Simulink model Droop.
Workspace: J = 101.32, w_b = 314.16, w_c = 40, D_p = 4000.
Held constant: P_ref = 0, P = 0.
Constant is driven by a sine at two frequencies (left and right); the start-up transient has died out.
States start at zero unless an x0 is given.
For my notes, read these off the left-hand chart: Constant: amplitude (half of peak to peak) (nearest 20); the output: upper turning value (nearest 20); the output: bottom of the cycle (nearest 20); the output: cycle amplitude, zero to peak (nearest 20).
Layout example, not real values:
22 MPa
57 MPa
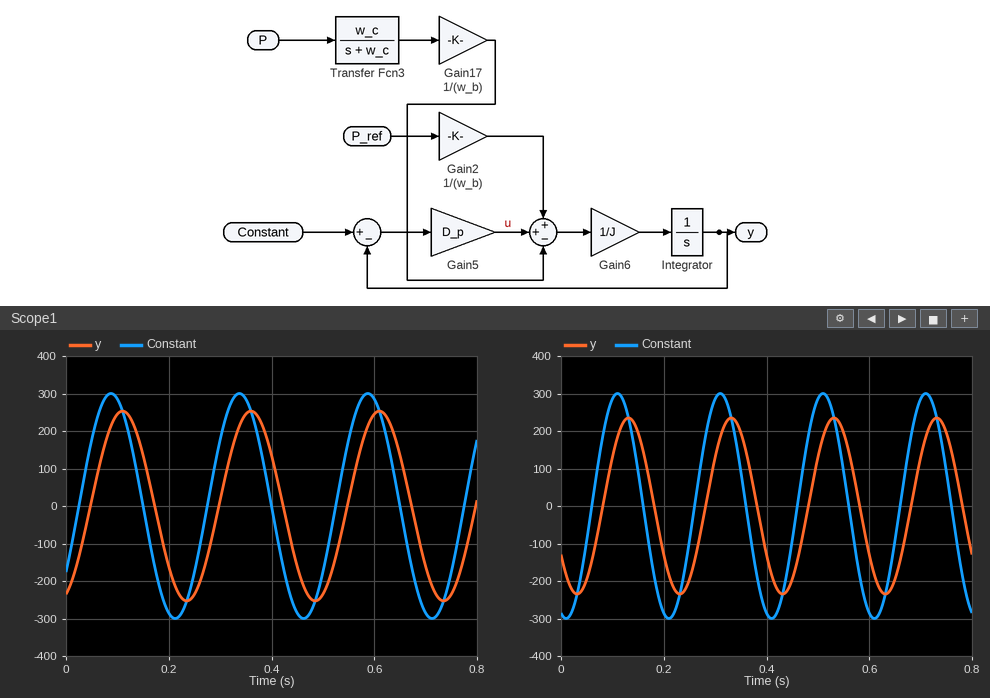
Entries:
300
260
-260
260
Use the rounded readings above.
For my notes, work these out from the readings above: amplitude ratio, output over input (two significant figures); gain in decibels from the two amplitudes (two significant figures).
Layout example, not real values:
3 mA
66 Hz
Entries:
0.87
-1.2 dB
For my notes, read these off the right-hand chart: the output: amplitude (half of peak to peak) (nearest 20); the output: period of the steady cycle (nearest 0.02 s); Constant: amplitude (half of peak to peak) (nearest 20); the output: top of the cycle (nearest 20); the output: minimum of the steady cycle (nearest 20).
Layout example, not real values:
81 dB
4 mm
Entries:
240
0.20 s
300
240
-240
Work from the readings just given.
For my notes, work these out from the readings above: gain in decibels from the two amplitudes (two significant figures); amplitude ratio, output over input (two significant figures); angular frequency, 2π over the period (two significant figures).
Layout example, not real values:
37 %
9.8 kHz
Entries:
-1.9 dB
0.80
31 rad/s
